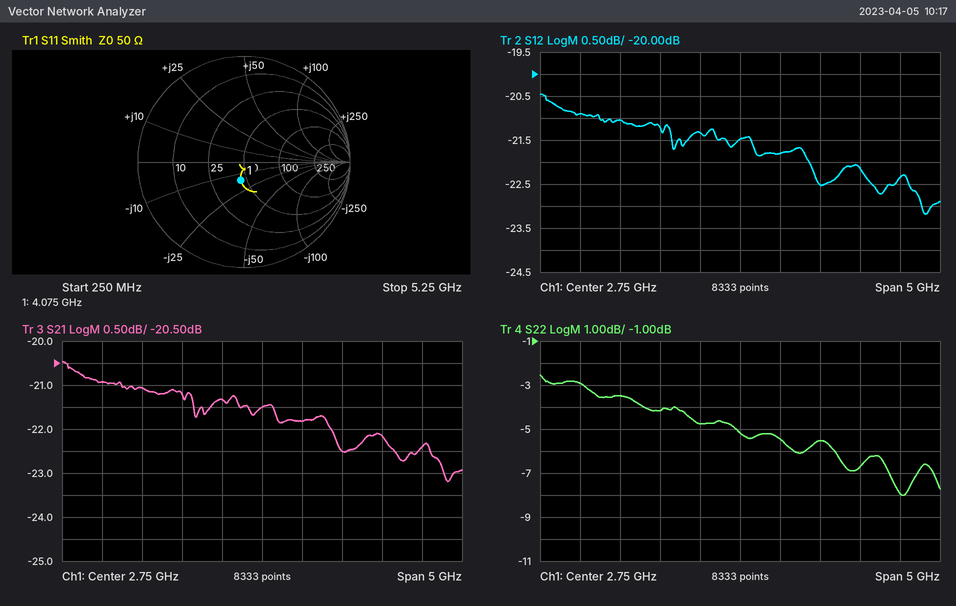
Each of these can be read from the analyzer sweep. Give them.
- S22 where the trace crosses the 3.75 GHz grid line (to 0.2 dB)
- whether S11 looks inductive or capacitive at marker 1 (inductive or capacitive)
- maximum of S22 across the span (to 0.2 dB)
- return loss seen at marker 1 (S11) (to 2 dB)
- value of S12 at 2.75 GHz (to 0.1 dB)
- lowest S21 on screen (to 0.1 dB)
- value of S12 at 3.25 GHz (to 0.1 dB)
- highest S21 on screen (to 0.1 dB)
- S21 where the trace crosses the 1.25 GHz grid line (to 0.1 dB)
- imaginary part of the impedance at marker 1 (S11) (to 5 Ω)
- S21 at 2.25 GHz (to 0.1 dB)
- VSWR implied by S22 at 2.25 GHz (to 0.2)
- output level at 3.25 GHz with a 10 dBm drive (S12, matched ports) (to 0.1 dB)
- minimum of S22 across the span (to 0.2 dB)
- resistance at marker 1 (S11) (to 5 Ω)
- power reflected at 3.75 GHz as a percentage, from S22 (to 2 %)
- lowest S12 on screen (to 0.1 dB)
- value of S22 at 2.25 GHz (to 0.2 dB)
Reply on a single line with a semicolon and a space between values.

-5.6 dB; capacitive; -2.6 dB; 16 dB; -21.5 dB; -23.2 dB; -21.8 dB; -20.5 dB; -21.1 dB; -15 Ω; -21.3 dB; 3.8; -11.8 dBm; -8.0 dB; 45 Ω; 28 %; -23.2 dB; -4.8 dB
